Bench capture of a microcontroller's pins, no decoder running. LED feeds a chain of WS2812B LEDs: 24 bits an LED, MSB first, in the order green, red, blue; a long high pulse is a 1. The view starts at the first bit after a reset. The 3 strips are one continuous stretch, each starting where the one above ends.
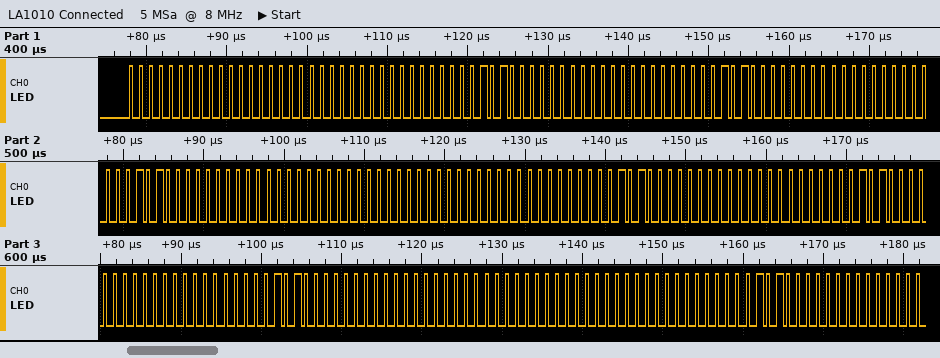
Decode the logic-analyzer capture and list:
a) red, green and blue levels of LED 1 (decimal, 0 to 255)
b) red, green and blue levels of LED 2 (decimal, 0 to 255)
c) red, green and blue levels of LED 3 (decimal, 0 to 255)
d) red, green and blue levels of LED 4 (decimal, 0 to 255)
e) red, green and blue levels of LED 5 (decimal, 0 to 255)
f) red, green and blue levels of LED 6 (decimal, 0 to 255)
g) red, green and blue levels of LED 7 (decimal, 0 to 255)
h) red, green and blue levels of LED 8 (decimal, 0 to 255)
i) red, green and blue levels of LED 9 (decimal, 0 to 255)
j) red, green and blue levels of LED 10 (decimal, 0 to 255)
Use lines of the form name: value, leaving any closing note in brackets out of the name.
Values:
red, green and blue levels of LED 1: 0, 0, 0
red, green and blue levels of LED 2: 20, 0, 0
red, green and blue levels of LED 3: 20, 0, 0
red, green and blue levels of LED 4: 20, 0, 0
red, green and blue levels of LED 5: 0, 0, 0
red, green and blue levels of LED 6: 20, 0, 0
red, green and blue levels of LED 7: 20, 0, 0
red, green and blue levels of LED 8: 20, 0, 0
red, green and blue levels of LED 9: 0, 0, 0
red, green and blue levels of LED 10: 20, 0, 0
